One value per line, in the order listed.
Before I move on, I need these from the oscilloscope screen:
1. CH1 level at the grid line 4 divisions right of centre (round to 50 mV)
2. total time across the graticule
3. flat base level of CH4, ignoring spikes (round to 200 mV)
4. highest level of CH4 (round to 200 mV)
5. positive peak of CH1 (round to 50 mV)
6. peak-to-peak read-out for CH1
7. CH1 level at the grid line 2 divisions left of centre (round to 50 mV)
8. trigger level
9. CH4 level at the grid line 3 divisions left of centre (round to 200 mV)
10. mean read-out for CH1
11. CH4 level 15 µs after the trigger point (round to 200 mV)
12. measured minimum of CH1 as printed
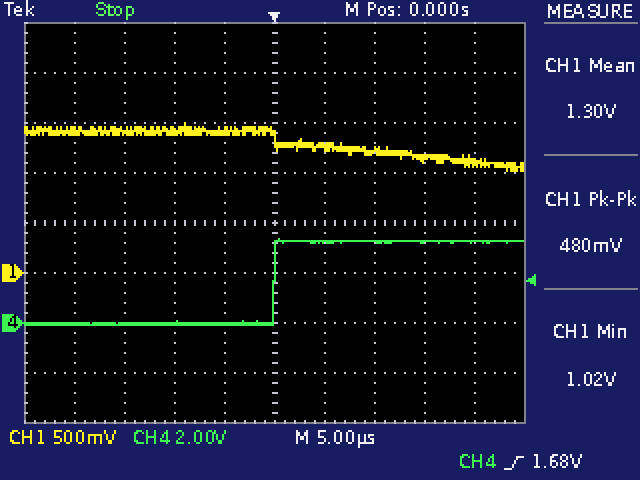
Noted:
1.10 V
50 µs
0.0 V
3.4 V
1.50 V
480 mV
1.40 V
1.68 V
0.0 V
1.30 V
3.2 V
1.02 V
